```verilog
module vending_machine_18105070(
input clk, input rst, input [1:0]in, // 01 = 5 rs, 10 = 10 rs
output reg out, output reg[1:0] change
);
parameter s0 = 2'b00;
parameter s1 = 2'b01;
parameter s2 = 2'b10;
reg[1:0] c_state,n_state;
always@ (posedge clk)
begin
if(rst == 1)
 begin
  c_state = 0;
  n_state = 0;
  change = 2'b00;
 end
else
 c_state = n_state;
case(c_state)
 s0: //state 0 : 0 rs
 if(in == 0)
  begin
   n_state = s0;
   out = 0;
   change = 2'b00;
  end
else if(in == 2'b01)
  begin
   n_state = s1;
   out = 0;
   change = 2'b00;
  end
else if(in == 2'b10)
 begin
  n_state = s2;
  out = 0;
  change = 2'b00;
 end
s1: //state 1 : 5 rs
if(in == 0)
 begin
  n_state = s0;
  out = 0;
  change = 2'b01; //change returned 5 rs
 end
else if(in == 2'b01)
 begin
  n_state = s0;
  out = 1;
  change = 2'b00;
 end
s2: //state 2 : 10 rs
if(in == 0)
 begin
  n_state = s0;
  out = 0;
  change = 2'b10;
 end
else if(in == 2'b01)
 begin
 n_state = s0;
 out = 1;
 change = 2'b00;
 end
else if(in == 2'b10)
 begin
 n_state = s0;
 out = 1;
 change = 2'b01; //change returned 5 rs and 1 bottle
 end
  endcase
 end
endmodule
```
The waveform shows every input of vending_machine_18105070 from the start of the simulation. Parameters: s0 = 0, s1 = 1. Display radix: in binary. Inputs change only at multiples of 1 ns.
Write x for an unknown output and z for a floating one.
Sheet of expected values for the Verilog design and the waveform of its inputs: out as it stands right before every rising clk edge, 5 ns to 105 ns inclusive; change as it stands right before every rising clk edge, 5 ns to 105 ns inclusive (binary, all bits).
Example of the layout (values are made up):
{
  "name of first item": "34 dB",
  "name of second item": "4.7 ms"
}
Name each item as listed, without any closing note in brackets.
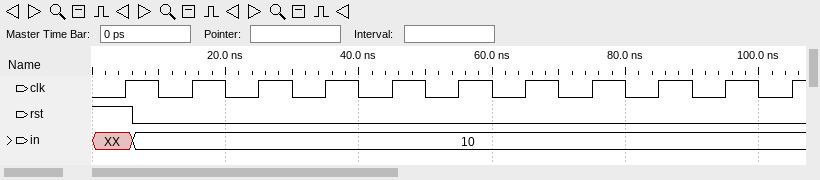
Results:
{
  "out as it stands right before every rising clk edge, 5 ns to 105 ns inclusive": "x x 0 1 0 1 0 1 0 1 0",
  "change as it stands right before every rising clk edge, 5 ns to 105 ns inclusive": "x, 00, 00, 01, 00, 01, 00, 01, 00, 01, 00"
}
